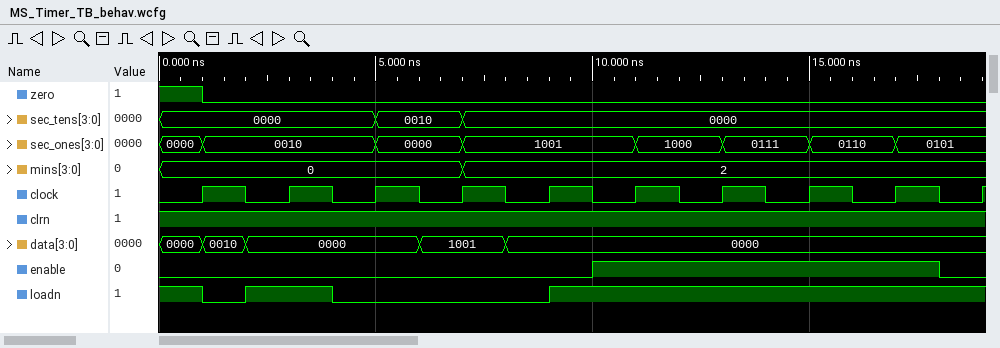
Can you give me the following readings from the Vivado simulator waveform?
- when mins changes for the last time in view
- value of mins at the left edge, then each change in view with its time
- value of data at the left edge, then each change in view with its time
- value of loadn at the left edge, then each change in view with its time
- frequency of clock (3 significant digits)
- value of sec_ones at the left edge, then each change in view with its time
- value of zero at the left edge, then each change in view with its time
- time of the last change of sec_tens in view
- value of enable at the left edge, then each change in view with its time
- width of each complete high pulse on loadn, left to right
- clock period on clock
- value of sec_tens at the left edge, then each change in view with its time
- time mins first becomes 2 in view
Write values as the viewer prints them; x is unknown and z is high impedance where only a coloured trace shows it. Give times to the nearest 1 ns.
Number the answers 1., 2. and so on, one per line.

1. 7 ns
2. 0, 2 at 7 ns
3. 0000, 0010 at 1 ns, 0000 at 2 ns, 1001 at 6 ns, 0000 at 8 ns
4. 1, 0 at 1 ns, 1 at 2 ns, 0 at 4 ns, 1 at 9 ns
5. 500 MHz
6. 0000, 0010 at 1 ns, 0000 at 5 ns, 1001 at 7 ns, 1000 at 11 ns, 0111 at 13 ns, 0110 at 15 ns, 0101 at 17 ns
7. 1, 0 at 1 ns
8. 7 ns
9. 0, 1 at 10 ns, 0 at 18 ns
10. 2 ns
11. 2 ns
12. 0000, 0010 at 5 ns, 0000 at 7 ns
13. 7 ns
